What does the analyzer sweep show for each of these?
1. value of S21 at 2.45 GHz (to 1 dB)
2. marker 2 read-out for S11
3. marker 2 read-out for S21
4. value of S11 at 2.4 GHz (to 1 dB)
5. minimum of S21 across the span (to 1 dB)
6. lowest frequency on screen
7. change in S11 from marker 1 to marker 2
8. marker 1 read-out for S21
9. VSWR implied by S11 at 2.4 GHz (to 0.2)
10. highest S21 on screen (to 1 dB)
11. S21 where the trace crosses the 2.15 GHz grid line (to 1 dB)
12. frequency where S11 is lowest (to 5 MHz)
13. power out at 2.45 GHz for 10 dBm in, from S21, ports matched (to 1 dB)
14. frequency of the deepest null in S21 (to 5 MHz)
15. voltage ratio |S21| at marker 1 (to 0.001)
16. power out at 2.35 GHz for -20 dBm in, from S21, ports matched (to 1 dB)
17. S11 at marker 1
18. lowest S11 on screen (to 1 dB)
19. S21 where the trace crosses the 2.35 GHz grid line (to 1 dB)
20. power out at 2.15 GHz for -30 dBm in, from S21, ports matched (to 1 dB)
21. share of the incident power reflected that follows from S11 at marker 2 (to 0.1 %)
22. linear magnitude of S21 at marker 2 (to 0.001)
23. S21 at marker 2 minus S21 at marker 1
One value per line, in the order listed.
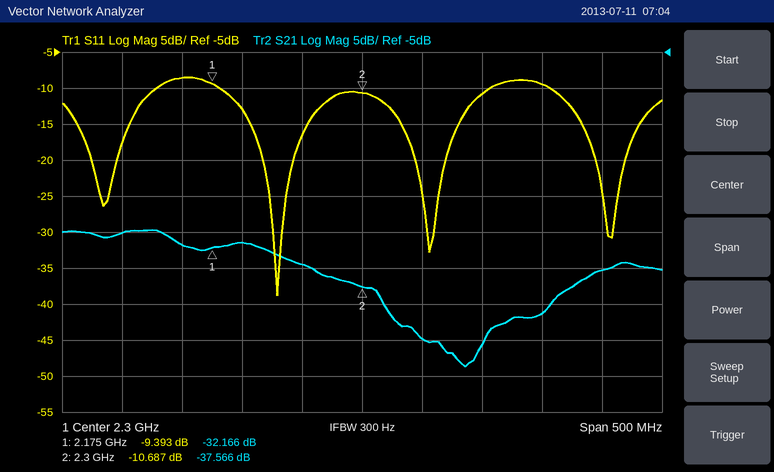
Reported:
-41 dB
-10.687 dB
-37.566 dB
-11 dB
-49 dB
2.05 GHz
-1.294 dB
-32.166 dB
1.8
-30 dB
-32 dB
2.230 GHz
-31 dBm
2.385 GHz
0.025
-65 dBm
-9.393 dB
-39 dB
-45 dB
-62 dBm
8.5 %
0.013
-5.400 dB
